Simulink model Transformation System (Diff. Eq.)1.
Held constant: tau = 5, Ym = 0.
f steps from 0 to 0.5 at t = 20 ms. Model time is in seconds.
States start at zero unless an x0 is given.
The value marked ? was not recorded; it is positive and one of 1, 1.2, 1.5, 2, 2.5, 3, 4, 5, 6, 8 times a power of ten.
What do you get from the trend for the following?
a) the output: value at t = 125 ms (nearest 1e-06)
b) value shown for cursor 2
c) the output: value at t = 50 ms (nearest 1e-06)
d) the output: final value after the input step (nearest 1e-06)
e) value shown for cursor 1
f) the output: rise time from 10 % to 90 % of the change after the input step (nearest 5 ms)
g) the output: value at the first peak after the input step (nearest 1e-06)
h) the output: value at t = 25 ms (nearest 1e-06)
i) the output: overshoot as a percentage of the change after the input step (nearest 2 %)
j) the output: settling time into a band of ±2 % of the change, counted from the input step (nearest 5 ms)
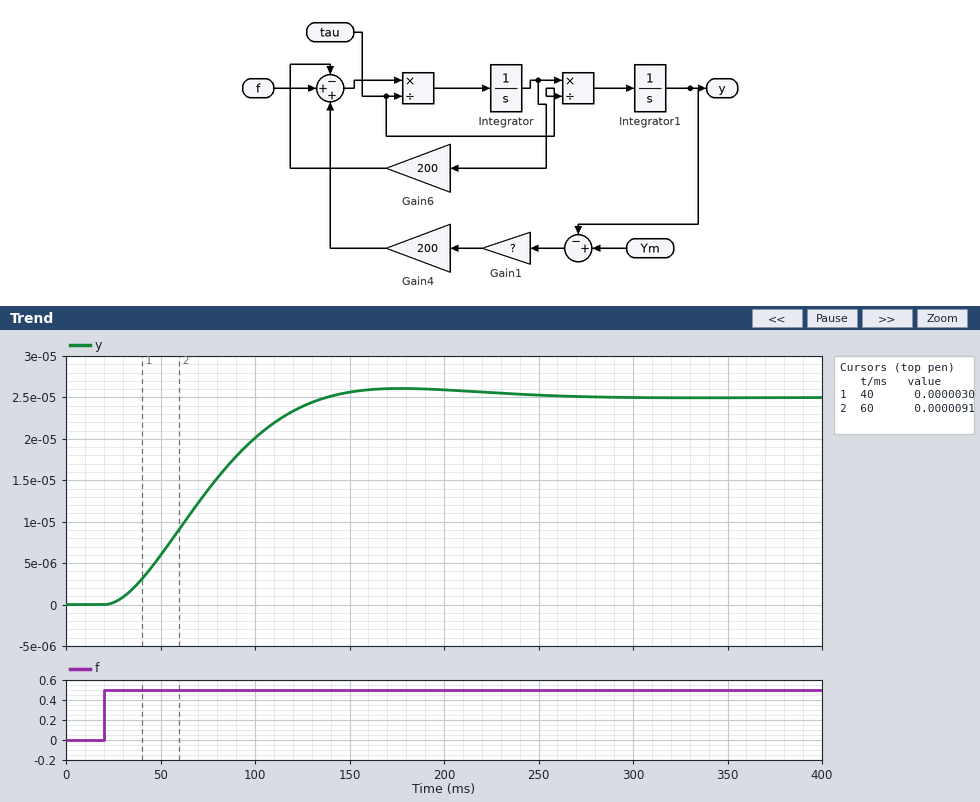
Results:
0.000024
0.0000091
0.000006
0.000025
0.0000030
75 ms
0.000026
0.000000
4 %
210 ms
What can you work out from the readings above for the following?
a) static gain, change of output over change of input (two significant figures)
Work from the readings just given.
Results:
0.000050
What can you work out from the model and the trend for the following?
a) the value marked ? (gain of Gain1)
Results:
100
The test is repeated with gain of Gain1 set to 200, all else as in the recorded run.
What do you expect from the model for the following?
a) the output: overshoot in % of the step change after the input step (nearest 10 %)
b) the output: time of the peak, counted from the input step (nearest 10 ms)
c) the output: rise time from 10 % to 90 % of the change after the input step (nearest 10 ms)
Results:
20 %
90 ms
40 ms
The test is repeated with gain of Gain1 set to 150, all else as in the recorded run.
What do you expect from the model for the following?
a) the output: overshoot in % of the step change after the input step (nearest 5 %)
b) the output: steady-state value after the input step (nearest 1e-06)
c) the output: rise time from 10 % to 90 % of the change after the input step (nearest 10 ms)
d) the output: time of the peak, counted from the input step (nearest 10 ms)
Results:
10 %
0.000017
50 ms
110 ms
